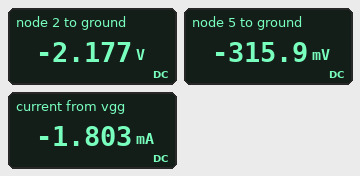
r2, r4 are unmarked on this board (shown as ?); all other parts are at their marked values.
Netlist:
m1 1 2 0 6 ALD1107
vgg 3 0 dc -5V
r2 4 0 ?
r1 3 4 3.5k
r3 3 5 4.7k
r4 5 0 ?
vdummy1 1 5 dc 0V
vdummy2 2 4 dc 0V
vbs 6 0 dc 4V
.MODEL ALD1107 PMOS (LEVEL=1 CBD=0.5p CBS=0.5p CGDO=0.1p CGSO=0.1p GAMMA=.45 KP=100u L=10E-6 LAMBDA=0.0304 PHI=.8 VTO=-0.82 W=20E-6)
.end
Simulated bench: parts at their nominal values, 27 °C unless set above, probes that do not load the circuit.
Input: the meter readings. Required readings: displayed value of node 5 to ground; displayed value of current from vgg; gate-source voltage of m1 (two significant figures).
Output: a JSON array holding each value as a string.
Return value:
["-315.9 mV", "-1.803 mA", "-2.2 V"]
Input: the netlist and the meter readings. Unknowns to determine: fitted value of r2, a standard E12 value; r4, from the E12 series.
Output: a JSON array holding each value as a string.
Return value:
["2.7 kΩ", "330 Ω"]
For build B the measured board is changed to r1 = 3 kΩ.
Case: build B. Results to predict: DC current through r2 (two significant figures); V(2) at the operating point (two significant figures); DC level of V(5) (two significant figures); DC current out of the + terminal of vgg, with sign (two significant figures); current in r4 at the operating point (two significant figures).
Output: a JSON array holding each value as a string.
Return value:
["880 µA", "-2.4 V", "-310 mV", "-1.9 mA", "950 µA"]
